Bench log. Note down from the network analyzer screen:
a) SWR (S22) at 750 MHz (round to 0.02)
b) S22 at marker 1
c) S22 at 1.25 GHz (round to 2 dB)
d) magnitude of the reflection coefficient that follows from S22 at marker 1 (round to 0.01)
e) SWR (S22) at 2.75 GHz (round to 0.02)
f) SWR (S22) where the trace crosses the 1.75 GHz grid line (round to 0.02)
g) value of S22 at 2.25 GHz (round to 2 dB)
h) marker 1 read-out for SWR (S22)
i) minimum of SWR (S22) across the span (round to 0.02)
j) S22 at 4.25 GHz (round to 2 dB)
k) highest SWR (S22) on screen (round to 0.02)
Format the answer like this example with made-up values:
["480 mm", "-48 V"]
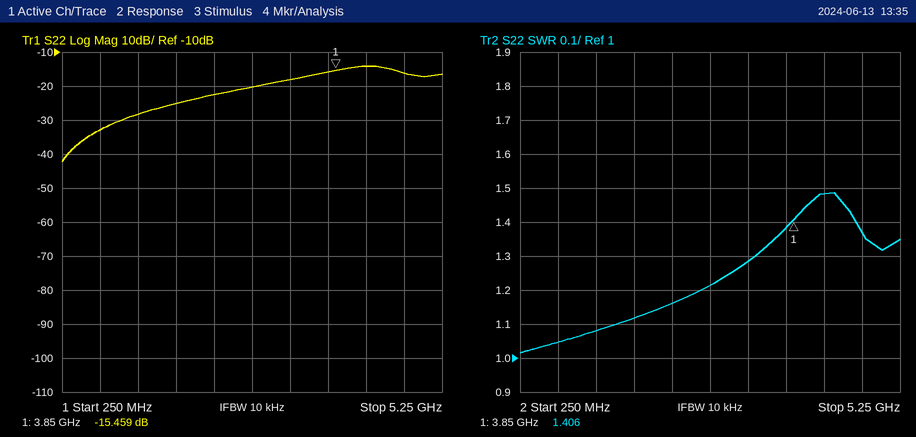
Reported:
["1.04", "-15.459 dB", "-28 dB", "0.17", "1.22", "1.12", "-22 dB", "1.406", "1.02", "-14 dB", "1.48"]
